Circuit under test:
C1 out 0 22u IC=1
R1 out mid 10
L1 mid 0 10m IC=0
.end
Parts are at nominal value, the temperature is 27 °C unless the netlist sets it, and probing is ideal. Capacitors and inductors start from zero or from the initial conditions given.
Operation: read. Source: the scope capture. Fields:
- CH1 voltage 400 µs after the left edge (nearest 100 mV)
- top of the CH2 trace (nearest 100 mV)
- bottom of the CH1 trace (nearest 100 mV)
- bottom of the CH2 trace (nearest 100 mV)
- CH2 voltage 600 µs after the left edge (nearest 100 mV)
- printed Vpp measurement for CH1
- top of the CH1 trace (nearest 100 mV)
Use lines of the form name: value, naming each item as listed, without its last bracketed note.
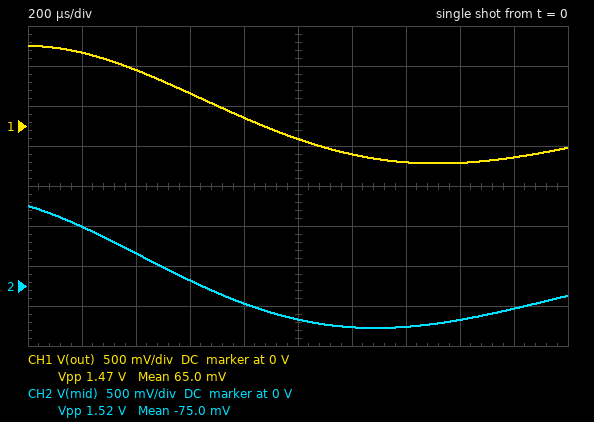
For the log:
CH1 voltage 400 µs after the left edge: 700 mV
top of the CH2 trace: 1.0 V
bottom of the CH1 trace: -500 mV
bottom of the CH2 trace: -500 mV
CH2 voltage 600 µs after the left edge: 100 mV
printed Vpp measurement for CH1: 1.47 V
top of the CH1 trace: 1.0 V
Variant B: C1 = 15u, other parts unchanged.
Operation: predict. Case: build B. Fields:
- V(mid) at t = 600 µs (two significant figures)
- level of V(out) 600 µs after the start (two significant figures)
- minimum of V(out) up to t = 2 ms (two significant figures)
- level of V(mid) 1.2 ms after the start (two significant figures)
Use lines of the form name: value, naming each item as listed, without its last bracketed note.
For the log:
V(mid) at t = 600 µs: -110 mV
level of V(out) 600 µs after the start: 180 mV
minimum of V(out) up to t = 2 ms: -540 mV
level of V(mid) 1.2 ms after the start: -560 mV
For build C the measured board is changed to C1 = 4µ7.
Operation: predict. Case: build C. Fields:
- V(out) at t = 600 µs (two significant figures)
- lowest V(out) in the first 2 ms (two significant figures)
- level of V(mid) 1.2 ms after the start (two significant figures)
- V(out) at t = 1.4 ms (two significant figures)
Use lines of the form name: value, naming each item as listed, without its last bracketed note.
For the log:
V(out) at t = 600 µs: -650 mV
lowest V(out) in the first 2 ms: -710 mV
level of V(mid) 1.2 ms after the start: 430 mV
V(out) at t = 1.4 ms: 500 mV
